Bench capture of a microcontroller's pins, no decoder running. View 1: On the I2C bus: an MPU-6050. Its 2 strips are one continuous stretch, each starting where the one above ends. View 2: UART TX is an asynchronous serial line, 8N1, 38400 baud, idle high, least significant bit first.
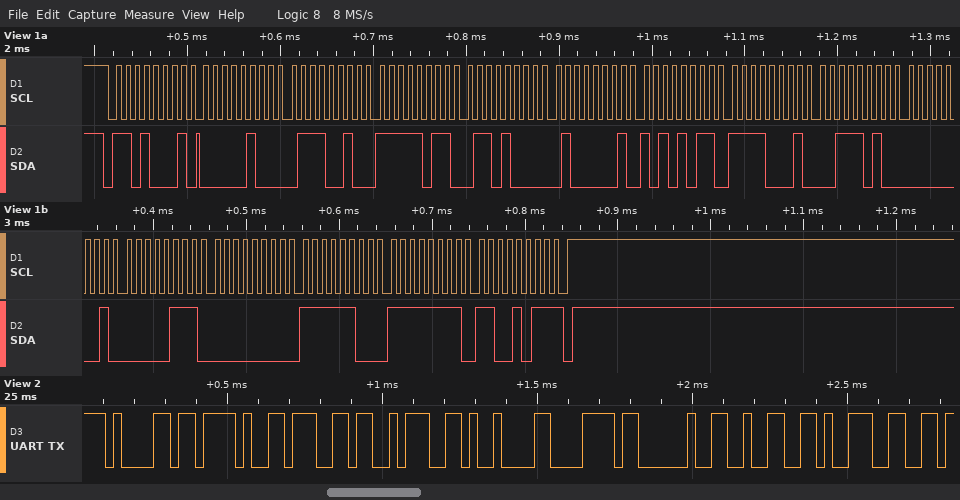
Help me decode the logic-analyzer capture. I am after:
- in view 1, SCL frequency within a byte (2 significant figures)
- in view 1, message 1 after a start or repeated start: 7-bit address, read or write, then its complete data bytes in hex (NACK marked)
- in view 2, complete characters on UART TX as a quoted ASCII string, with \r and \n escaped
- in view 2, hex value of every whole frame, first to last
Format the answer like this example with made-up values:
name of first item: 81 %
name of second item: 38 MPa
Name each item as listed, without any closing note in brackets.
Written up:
in view 1, SCL frequency within a byte: 100 kHz
in view 1, message 1 after a start or repeated start: 7-bit address, read or write, then its complete data bytes in hex: 0x68 read: 04 72 FB 68 41 AB F1 3A 01 07 00 FC FF CB NACK
in view 2, complete characters on UART TX as a quoted ASCII string, with \r and \n escaped: "a/g:\tx 29"
in view 2, hex value of every whole frame, first to last: 61 2F 67 3A 09 78 20 32 39
